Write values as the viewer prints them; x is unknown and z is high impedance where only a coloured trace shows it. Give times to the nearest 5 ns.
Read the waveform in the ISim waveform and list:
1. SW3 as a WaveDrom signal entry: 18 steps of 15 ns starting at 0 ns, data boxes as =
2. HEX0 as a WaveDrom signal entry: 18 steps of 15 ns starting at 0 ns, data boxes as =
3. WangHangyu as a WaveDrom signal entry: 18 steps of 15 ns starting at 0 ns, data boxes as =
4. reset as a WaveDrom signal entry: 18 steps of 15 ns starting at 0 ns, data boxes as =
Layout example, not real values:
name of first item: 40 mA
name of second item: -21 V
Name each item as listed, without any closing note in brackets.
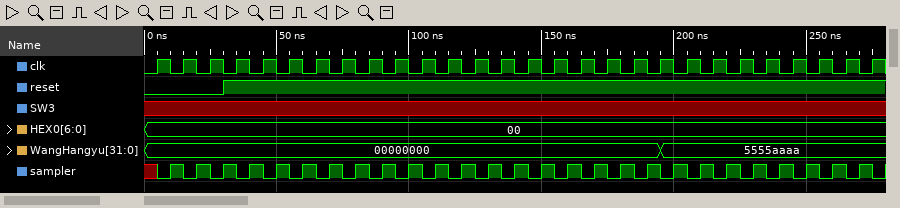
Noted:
SW3 as a WaveDrom signal entry: 18 steps of 15 ns starting at 0 ns, data boxes as =: {name: 'SW3', wave: 'x.................'}
HEX0 as a WaveDrom signal entry: 18 steps of 15 ns starting at 0 ns, data boxes as =: {name: 'HEX0', wave: '=.................', data: '00'}
WangHangyu as a WaveDrom signal entry: 18 steps of 15 ns starting at 0 ns, data boxes as =: {name: 'WangHangyu', wave: '=............=....', data: '00000000 5555aaaa'}
reset as a WaveDrom signal entry: 18 steps of 15 ns starting at 0 ns, data boxes as =: {name: 'reset', wave: '0.1...............'}
